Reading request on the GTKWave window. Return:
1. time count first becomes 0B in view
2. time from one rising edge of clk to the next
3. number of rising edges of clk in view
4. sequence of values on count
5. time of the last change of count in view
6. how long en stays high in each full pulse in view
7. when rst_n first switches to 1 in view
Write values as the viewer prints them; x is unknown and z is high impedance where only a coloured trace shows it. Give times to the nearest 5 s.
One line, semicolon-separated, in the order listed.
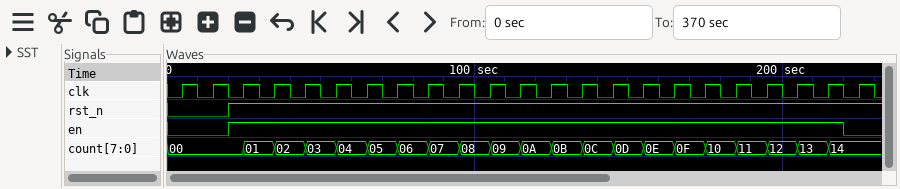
125 s; 10 s; 23; 00, 01, 02, 03, 04, 05, 06, 07, 08, 09, 0A, 0B, 0C, 0D, 0E, 0F, 10, 11, 12, 13, 14; 215 s; 200 s; 20 s
